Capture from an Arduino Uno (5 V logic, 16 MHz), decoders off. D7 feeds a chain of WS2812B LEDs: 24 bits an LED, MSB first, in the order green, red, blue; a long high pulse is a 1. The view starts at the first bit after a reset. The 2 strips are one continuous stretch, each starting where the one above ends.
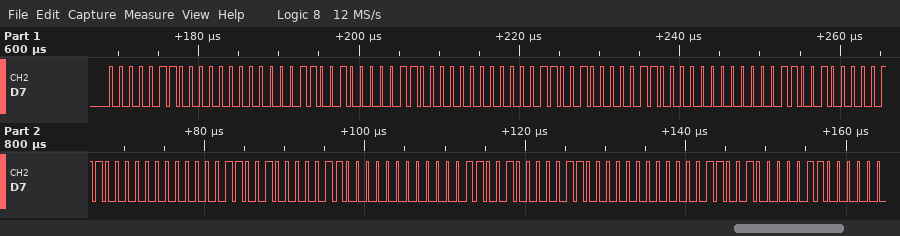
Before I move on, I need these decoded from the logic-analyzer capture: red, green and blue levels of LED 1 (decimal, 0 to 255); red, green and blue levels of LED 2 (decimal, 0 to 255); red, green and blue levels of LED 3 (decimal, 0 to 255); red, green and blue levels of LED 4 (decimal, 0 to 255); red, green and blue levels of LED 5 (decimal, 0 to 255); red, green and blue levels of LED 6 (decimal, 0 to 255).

0, 6, 25
0, 6, 25
0, 6, 25
0, 6, 25
0, 6, 25
0, 6, 25
